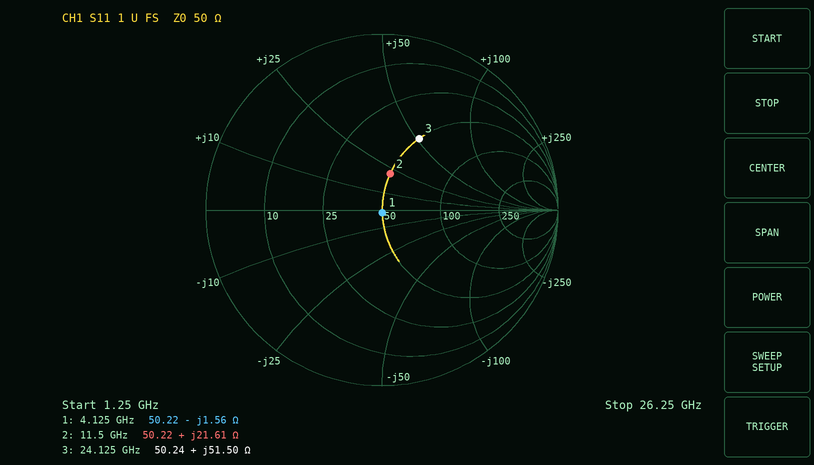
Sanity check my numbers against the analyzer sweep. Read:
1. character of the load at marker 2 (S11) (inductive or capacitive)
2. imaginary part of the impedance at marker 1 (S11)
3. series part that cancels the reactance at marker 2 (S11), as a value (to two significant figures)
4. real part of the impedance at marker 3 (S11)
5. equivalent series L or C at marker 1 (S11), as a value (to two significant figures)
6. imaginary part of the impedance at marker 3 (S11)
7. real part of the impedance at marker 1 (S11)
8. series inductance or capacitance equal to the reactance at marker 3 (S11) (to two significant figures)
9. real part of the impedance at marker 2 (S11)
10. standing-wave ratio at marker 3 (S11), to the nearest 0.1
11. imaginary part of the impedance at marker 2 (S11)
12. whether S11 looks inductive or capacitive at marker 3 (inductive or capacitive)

inductive
-1.56 Ω
640 fF
50.24 Ω
25 pF
+51.50 Ω
50.22 Ω
340 pH
50.22 Ω
2.7
+21.61 Ω
inductive
